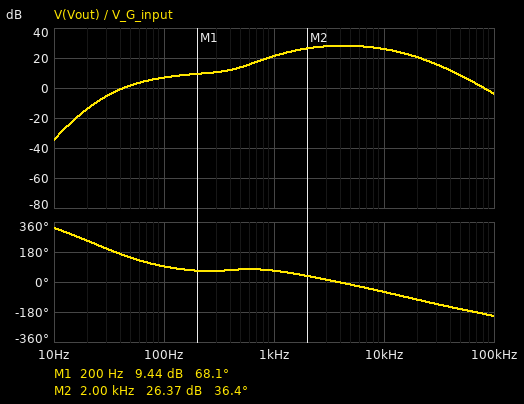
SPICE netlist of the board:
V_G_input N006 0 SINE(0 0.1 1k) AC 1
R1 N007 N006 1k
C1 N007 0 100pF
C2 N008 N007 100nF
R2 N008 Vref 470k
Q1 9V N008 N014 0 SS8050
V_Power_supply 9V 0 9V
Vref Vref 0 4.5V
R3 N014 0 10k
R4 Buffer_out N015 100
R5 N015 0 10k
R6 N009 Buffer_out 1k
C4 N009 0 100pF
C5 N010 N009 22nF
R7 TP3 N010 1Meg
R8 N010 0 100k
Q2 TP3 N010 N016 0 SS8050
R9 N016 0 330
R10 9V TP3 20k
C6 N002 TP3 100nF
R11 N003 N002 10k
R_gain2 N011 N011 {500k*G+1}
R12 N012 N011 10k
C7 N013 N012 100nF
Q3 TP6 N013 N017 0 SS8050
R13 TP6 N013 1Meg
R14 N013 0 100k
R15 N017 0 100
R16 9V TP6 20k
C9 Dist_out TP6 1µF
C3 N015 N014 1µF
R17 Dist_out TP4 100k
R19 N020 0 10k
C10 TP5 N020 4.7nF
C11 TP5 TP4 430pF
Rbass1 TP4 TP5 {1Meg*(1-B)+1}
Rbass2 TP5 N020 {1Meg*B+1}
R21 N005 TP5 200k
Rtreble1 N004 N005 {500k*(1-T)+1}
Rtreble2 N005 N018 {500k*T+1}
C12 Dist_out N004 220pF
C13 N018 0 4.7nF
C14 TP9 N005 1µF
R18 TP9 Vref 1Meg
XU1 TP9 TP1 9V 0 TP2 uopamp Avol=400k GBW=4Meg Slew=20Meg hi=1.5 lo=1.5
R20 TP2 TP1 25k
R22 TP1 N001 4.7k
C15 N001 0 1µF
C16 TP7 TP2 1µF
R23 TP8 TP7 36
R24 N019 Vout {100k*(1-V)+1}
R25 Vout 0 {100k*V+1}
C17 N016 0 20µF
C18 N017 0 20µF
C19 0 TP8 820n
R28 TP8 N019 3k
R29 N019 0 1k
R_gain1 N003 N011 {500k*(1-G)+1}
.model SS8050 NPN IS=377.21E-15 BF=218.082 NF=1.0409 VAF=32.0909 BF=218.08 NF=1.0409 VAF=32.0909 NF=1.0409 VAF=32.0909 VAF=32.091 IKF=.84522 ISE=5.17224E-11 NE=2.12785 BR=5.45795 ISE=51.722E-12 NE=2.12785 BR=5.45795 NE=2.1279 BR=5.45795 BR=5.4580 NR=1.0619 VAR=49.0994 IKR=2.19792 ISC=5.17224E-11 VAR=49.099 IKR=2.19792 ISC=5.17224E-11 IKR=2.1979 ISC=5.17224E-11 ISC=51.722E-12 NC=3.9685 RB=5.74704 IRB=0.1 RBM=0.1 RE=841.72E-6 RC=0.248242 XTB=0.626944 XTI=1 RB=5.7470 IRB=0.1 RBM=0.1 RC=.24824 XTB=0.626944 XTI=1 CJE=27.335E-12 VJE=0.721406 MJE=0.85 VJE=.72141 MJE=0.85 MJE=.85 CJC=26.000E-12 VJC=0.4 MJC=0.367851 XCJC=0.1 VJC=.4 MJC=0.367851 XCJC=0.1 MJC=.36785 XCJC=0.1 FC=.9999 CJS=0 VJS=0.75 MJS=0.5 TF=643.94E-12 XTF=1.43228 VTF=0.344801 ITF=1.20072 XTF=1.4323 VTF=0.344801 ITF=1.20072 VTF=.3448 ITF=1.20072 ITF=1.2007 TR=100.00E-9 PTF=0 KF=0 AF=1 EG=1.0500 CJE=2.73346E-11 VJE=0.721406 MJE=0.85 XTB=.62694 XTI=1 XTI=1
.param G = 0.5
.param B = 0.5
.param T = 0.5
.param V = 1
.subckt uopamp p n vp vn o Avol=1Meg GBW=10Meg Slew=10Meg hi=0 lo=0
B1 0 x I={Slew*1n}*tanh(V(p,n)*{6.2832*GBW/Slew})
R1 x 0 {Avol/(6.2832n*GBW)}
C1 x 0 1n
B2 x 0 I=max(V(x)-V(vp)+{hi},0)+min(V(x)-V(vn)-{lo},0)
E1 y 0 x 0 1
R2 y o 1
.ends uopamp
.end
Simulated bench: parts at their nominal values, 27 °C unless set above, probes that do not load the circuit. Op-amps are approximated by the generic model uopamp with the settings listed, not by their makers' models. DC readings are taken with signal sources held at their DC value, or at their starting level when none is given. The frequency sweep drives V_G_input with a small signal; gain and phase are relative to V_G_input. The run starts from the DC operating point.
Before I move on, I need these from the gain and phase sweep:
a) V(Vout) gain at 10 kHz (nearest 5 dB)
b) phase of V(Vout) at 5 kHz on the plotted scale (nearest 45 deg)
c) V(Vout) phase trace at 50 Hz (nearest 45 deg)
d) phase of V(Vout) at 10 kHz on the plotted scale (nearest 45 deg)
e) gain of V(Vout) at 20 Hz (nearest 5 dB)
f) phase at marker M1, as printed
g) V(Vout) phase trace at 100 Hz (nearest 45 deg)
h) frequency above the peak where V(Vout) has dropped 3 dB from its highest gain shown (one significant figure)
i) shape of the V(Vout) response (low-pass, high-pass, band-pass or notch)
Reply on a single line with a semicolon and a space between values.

25 dB; 0 deg; 135 deg; -45 deg; -15 dB; 68.1 deg; 90 deg; 10 kHz; band-pass
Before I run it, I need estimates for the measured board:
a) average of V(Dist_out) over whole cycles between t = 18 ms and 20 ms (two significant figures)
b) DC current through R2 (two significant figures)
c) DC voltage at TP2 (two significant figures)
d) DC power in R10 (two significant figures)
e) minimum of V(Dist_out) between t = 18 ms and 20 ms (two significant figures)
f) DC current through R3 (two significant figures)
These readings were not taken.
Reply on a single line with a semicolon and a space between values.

-1.5 V; 2.2 µA; 4.5 V; 200 µW; -4.3 V; 290 µA
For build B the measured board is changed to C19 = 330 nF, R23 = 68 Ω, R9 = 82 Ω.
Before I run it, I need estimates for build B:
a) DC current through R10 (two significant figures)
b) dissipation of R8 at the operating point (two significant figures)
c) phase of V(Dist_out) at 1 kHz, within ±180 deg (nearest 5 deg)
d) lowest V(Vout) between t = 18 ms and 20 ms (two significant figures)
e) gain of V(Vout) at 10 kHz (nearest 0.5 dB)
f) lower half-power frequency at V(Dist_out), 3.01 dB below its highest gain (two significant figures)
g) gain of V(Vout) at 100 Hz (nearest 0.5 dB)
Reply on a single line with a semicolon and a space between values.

110 µA; 2.8 µW; 35 deg; -410 mV; 29.0 dB; 620 Hz; 9.5 dB
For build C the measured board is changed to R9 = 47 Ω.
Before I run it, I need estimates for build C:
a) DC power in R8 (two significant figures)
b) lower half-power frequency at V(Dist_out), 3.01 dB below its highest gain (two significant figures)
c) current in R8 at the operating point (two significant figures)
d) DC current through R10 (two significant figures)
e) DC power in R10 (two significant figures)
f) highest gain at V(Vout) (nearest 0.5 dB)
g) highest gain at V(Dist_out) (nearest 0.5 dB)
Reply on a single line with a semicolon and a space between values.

2.7 µW; 620 Hz; 5.2 µA; 110 µA; 240 µW; 29.0 dB; 42.0 dB
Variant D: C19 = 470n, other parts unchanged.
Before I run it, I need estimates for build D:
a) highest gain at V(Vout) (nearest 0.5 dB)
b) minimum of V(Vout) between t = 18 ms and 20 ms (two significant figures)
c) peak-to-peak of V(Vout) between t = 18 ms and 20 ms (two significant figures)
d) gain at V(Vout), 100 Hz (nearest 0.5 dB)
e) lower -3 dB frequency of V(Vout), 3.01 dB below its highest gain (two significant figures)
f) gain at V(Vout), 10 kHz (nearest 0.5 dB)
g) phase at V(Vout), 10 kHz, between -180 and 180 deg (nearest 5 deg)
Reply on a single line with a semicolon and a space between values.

30.5 dB; -390 mV; 1.0 V; 8.5 dB; 1.7 kHz; 29.0 dB; -50 deg
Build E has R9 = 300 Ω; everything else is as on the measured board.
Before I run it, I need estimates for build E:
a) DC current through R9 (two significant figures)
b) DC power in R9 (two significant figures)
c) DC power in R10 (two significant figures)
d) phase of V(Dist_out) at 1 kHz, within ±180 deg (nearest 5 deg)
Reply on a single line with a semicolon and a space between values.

96 µA; 2.8 µW; 210 µW; 30 deg
